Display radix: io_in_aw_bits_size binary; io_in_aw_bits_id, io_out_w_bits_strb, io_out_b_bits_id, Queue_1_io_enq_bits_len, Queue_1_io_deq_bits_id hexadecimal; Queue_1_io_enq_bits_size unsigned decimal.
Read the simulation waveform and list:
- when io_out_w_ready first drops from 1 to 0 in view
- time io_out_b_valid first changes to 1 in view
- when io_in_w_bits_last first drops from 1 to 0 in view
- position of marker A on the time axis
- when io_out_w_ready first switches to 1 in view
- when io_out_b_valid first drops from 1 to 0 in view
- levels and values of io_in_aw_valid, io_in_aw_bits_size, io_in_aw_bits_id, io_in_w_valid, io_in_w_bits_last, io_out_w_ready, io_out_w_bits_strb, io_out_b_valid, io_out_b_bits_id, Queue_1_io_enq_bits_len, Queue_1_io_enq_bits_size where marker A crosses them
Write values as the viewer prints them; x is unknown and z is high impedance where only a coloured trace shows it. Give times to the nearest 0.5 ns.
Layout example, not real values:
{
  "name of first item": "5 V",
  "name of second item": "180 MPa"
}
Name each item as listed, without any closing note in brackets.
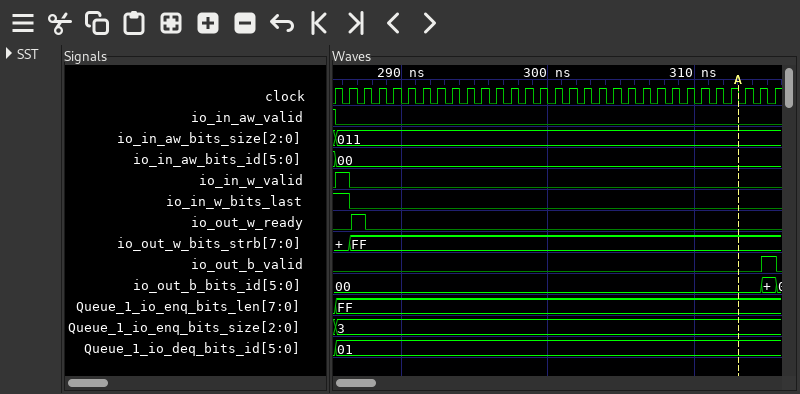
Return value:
{
  "when io_out_w_ready first drops from 1 to 0 in view": "287.5 ns",
  "time io_out_b_valid first changes to 1 in view": "314.5 ns",
  "when io_in_w_bits_last first drops from 1 to 0 in view": "286.5 ns",
  "position of marker A on the time axis": "313 ns",
  "when io_out_w_ready first switches to 1 in view": "286.5 ns",
  "when io_out_b_valid first drops from 1 to 0 in view": "315.5 ns",
  "levels and values of io_in_aw_valid, io_in_aw_bits_size, io_in_aw_bits_id, io_in_w_valid, io_in_w_bits_last, io_out_w_ready, io_out_w_bits_strb, io_out_b_valid, io_out_b_bits_id, Queue_1_io_enq_bits_len, Queue_1_io_enq_bits_size where marker A crosses them": "io_in_aw_valid=0, io_in_aw_bits_size=011, io_in_aw_bits_id=00, io_in_w_valid=0, io_in_w_bits_last=0, io_out_w_ready=0, io_out_w_bits_strb=FF, io_out_b_valid=0, io_out_b_bits_id=00, Queue_1_io_enq_bits_len=FF, Queue_1_io_enq_bits_size=3"
}
